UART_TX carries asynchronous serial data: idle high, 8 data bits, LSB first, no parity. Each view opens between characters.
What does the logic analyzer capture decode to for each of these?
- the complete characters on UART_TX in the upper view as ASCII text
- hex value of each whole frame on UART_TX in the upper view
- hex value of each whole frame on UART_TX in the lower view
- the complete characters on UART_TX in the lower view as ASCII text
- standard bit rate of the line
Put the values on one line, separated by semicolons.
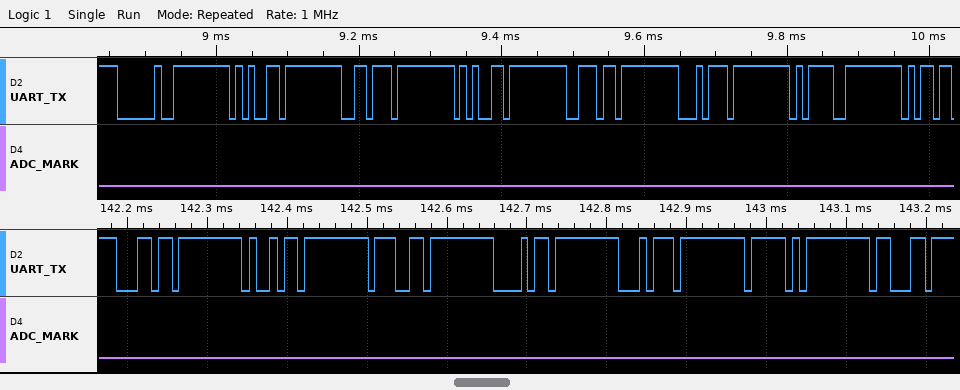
" event="; 20, 65, 76, 65, 6E, 74, 3D; 6C, 69, 67, 68, 74, 5F, 63; "light_c"; 115200 baud
